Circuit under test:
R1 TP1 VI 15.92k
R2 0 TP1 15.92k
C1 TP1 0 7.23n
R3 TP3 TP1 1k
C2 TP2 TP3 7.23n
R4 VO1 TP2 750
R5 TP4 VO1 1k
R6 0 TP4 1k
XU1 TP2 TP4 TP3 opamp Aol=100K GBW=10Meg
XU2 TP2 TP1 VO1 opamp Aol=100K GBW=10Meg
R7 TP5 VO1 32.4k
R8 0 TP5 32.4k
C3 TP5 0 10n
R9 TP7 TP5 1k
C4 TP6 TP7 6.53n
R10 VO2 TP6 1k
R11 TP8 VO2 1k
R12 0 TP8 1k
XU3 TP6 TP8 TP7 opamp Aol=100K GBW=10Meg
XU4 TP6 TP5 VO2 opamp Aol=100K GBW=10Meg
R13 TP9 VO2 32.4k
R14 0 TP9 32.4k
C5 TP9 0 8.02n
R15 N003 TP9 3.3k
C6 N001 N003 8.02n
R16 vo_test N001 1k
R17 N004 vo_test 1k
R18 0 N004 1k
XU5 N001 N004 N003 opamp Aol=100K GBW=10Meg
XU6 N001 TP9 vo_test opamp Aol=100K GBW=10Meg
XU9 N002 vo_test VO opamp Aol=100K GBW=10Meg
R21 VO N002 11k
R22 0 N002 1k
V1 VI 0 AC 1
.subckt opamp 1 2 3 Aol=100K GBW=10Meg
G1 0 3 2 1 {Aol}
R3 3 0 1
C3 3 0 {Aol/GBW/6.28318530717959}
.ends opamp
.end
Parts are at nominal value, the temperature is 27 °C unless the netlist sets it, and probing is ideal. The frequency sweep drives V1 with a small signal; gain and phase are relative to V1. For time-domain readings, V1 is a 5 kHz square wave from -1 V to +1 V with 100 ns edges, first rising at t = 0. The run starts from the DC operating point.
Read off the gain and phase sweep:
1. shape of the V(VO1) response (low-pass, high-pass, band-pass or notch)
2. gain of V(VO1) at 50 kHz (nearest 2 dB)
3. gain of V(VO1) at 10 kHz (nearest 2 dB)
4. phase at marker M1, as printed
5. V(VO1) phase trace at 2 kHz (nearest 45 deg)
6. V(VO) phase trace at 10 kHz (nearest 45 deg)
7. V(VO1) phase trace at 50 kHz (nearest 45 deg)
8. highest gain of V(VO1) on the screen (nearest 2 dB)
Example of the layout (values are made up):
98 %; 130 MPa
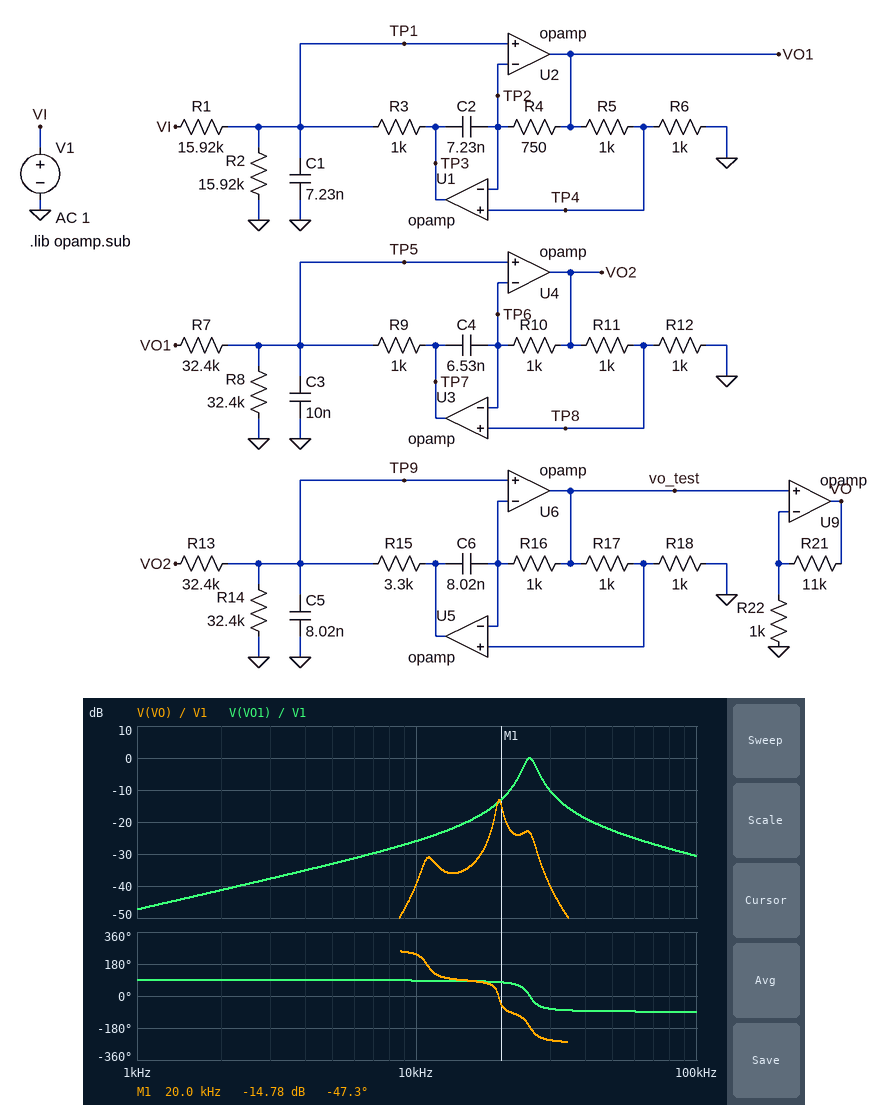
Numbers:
band-pass; -22 dB; -26 dB; -47.3 deg; 90 deg; 225 deg; -90 deg; 0 dB
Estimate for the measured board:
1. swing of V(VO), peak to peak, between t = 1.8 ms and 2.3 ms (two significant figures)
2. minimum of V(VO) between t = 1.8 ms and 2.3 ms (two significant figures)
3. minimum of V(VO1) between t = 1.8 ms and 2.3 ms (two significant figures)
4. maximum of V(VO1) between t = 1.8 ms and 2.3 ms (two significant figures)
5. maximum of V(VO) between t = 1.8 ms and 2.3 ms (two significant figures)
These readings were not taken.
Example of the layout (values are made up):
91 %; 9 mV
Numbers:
51 mV; -26 mV; -340 mV; 340 mV; 26 mV
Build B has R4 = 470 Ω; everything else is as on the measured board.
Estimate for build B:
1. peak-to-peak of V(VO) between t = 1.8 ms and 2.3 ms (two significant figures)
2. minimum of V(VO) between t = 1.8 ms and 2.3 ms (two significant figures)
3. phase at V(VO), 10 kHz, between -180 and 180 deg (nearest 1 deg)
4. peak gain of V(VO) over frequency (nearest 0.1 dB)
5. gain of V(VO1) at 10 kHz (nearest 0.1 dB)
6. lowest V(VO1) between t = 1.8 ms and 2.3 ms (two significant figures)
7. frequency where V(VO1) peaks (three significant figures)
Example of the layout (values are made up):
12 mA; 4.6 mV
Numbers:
16 mV; -8.0 mV; -128 deg; -20.8 dB; -30.5 dB; -130 mV; 31.9 kHz
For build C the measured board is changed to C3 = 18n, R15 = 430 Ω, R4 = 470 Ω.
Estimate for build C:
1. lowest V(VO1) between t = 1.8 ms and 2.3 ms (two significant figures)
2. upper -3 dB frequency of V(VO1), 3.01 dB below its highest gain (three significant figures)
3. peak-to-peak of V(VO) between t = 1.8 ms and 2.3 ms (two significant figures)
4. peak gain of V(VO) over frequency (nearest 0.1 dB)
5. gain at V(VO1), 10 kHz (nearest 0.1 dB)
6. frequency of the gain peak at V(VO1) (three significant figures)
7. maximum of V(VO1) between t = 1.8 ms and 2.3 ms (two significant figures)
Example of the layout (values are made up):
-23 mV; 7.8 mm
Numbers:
-130 mV; 33.3 kHz; 16 mV; -15.4 dB; -30.5 dB; 31.9 kHz; 130 mV
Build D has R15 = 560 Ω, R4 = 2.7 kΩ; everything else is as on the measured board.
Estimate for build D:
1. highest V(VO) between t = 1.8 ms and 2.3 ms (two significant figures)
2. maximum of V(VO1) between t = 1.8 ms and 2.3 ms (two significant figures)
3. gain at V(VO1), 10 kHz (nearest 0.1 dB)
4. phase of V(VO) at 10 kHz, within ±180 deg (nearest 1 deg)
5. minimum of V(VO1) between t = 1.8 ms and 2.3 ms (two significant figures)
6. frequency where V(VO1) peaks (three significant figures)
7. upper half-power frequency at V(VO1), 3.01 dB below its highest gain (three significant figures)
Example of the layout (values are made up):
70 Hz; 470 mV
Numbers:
31 mV; 380 mV; -9.6 dB; -113 deg; -380 mV; 13.4 kHz; 14.8 kHz
